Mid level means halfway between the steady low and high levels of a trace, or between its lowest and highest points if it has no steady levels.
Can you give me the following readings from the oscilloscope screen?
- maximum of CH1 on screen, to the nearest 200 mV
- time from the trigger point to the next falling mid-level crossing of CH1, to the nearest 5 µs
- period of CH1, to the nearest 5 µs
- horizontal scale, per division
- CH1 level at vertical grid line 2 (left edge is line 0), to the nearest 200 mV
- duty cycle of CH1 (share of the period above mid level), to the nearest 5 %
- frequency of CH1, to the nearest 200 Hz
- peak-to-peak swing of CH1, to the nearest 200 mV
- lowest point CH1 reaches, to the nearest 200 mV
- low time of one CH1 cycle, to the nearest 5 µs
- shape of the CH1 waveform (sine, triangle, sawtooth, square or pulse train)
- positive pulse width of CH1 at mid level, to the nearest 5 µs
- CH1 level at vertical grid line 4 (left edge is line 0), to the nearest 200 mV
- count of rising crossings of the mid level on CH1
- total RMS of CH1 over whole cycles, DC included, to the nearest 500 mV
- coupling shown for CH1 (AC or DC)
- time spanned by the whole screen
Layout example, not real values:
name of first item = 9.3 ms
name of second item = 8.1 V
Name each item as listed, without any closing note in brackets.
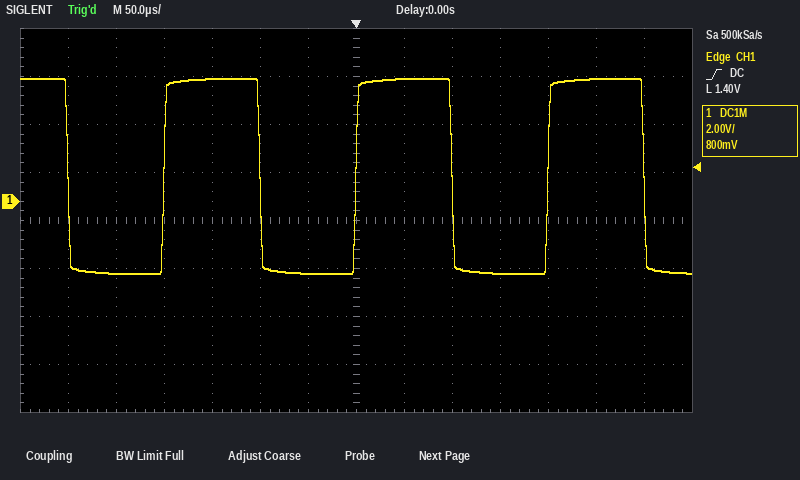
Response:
maximum of CH1 on screen, to the nearest 200 mV = 5.2 V
time from the trigger point to the next falling mid-level crossing of CH1, to the nearest 5 µs = 100 µs
period of CH1, to the nearest 5 µs = 200 µs
horizontal scale, per division = 50 µs
CH1 level at vertical grid line 2 (left edge is line 0), to the nearest 200 mV = -3.0 V
duty cycle of CH1 (share of the period above mid level), to the nearest 5 % = 50 %
frequency of CH1, to the nearest 200 Hz = 5.0 kHz
peak-to-peak swing of CH1, to the nearest 200 mV = 8.2 V
lowest point CH1 reaches, to the nearest 200 mV = -3.0 V
low time of one CH1 cycle, to the nearest 5 µs = 100 µs
shape of the CH1 waveform = square
positive pulse width of CH1 at mid level, to the nearest 5 µs = 100 µs
CH1 level at vertical grid line 4 (left edge is line 0), to the nearest 200 mV = 5.2 V
count of rising crossings of the mid level on CH1 = 3
total RMS of CH1 over whole cycles, DC included, to the nearest 500 mV = 4.0 V
coupling shown for CH1 = DC
time spanned by the whole screen = 700 µs
